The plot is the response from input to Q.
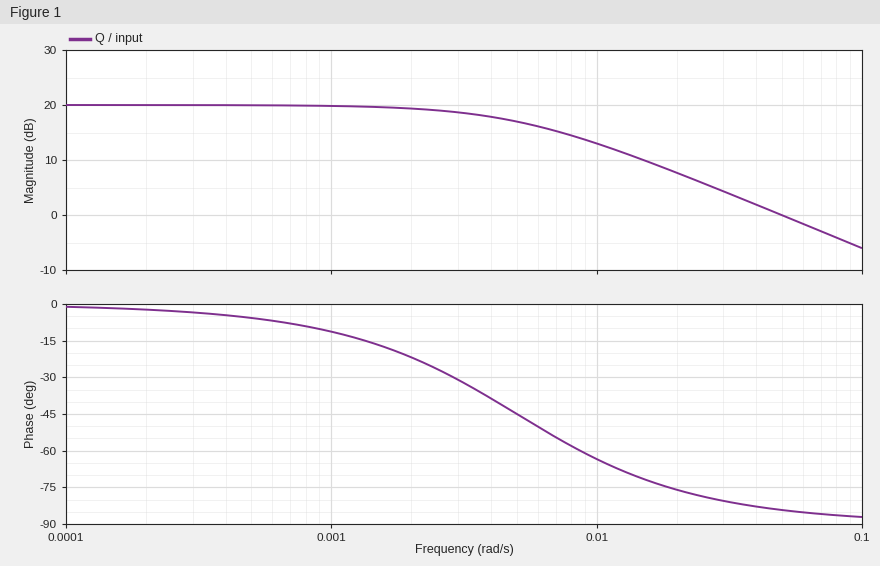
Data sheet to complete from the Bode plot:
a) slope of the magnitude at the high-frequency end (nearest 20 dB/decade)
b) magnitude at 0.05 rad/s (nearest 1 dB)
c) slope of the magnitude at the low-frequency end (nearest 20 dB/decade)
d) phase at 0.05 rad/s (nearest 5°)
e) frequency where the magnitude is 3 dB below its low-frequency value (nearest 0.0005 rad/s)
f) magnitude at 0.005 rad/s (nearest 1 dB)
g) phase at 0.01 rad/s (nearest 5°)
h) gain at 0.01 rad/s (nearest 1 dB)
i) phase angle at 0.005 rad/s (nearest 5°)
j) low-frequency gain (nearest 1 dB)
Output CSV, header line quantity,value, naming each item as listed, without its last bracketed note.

quantity,value
slope of the magnitude at the high-frequency end,-20 dB/decade
magnitude at 0.05 rad/s,0 dB
slope of the magnitude at the low-frequency end,0 dB/decade
phase at 0.05 rad/s,-85°
frequency where the magnitude is 3 dB below its low-frequency value,0.0050 rad/s
magnitude at 0.005 rad/s,17 dB
phase at 0.01 rad/s,-65°
gain at 0.01 rad/s,13 dB
phase angle at 0.005 rad/s,-45°
low-frequency gain,20 dB
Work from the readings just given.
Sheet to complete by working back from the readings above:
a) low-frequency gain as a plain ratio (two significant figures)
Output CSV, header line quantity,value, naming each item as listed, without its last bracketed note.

quantity,value
low-frequency gain as a plain ratio,10
